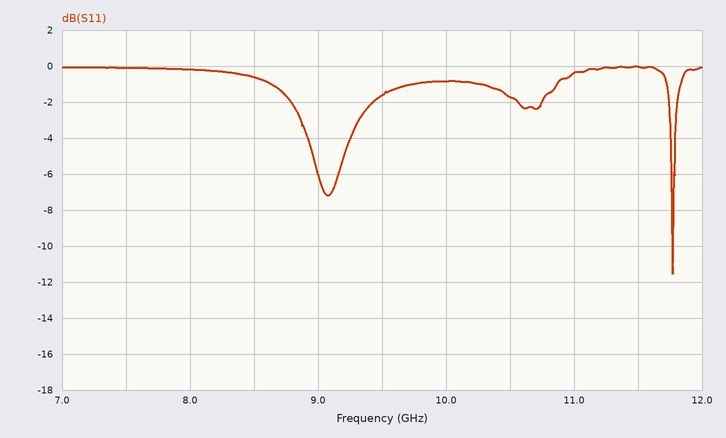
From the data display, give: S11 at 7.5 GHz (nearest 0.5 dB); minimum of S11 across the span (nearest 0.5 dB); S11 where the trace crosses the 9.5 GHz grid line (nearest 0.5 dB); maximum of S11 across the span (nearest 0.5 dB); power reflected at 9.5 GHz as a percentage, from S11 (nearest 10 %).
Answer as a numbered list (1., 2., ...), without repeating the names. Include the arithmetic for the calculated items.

1. 0.0 dB
2. -11.5 dB
3. -1.5 dB
4. 0.0 dB
5. 10^(-1.5/10) ≈ 70.8 %, so 70 % to the nearest 10 %
